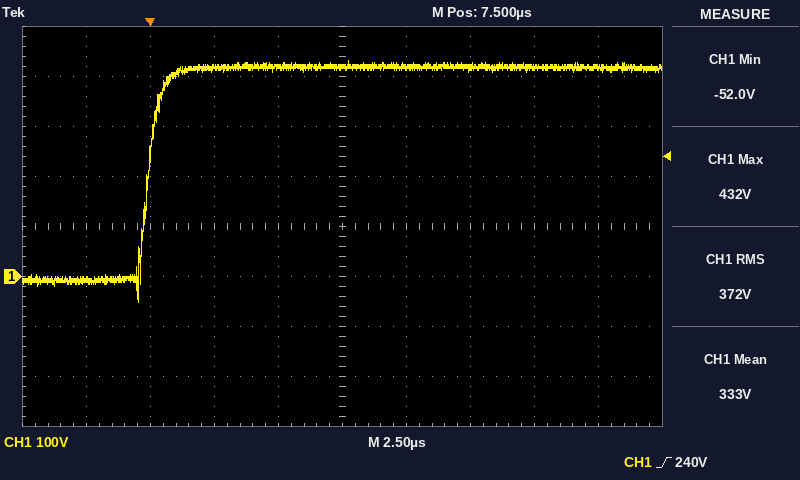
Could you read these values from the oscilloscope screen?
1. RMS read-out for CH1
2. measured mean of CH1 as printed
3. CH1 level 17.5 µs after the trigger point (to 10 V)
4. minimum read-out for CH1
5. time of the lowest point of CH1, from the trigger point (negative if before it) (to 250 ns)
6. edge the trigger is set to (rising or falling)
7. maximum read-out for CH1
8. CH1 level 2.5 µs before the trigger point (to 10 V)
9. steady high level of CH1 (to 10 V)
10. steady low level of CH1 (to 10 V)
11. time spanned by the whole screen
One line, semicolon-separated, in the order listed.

372 V; 333 V; 420 V; -52.0 V; -500 ns; rising; 432 V; -10 V; 420 V; -10 V; 25 µs
